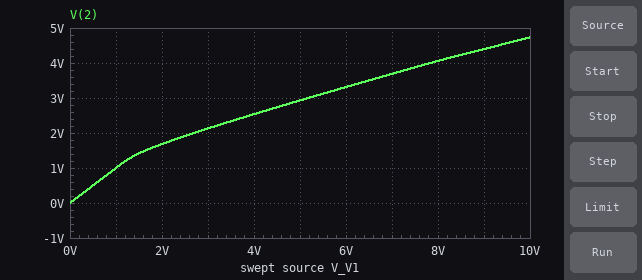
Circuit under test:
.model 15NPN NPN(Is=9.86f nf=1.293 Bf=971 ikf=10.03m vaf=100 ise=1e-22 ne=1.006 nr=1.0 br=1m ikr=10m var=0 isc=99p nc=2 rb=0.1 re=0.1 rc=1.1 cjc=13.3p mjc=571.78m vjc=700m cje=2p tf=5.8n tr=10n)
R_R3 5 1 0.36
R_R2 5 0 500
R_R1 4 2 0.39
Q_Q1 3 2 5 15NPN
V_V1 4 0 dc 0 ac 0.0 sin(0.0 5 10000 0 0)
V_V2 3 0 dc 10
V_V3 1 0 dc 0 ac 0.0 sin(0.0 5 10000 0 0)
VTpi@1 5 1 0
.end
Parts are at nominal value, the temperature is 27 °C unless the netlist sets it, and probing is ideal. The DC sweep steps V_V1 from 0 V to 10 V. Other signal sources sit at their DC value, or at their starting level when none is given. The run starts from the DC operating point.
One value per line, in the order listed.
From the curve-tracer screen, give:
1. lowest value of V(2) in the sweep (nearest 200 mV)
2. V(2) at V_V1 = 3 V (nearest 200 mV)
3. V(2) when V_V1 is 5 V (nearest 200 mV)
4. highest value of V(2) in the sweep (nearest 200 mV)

0 V
2.2 V
3.0 V
4.8 V
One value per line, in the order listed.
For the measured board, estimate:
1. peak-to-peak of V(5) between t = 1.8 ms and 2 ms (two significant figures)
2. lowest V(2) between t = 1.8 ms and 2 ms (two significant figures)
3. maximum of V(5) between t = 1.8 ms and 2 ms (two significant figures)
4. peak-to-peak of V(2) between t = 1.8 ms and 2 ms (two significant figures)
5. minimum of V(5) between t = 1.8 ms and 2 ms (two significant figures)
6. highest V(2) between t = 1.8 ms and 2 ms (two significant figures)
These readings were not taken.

10 V
-5.0 V
5.0 V
10 V
-5.0 V
5.0 V
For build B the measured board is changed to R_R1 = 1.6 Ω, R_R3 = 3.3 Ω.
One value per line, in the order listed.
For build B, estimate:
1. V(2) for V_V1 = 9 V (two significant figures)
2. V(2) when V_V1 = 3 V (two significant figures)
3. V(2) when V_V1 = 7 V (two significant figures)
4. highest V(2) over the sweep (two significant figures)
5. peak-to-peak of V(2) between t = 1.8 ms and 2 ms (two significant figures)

2.6 V
1.7 V
2.3 V
2.7 V
10 V
